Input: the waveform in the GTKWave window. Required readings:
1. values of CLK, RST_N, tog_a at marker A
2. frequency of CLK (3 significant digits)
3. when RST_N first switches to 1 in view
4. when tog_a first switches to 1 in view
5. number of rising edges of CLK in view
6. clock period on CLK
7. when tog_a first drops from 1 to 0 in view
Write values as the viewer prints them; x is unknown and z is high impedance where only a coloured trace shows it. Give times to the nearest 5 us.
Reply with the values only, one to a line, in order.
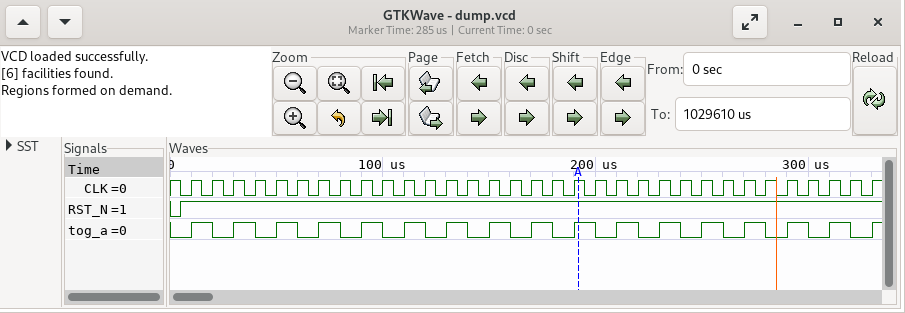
CLK=1, RST_N=1, tog_a=1
100 kHz
5 us
10 us
33
10 us
20 us
